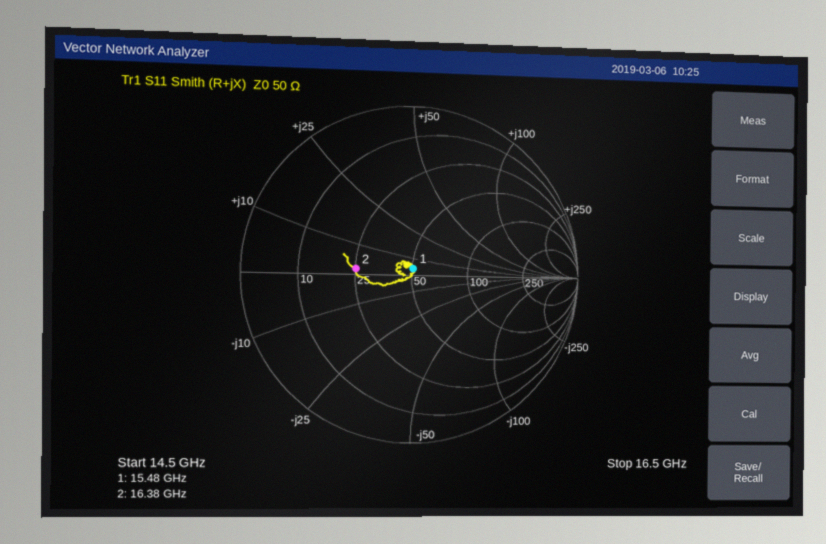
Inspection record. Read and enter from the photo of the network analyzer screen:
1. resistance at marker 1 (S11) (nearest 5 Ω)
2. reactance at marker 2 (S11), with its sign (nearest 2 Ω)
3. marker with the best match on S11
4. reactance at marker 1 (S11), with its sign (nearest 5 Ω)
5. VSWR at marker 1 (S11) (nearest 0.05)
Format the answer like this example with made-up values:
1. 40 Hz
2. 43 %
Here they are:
1. 50 Ω
2. +2 Ω
3. marker 1
4. +5 Ω
5. 1.10
